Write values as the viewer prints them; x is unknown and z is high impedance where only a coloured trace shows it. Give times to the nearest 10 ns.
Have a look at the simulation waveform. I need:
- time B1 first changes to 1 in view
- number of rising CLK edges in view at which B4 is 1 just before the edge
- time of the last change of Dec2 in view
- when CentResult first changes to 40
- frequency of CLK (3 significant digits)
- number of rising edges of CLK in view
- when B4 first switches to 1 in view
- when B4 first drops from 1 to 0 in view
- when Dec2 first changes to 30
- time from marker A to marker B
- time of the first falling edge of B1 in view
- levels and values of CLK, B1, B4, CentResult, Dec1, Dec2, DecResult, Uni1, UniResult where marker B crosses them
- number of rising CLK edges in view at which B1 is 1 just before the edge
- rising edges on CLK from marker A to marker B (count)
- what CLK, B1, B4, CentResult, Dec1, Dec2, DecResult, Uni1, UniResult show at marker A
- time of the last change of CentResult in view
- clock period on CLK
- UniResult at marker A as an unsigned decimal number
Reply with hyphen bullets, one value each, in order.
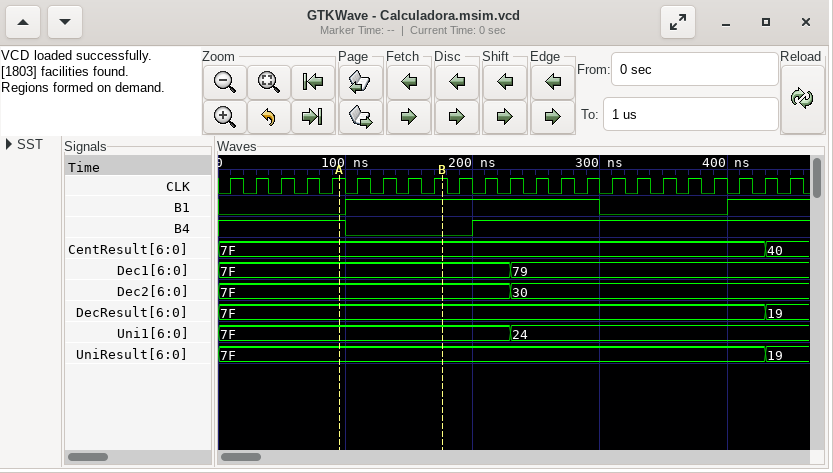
- 100 ns
- 18
- 230 ns
- 430 ns
- 50.0 MHz
- 23
- 200 ns
- 100 ns
- 230 ns
- 80 ns
- 300 ns
- CLK=1, B1=1, B4=0, CentResult=7F, Dec1=7F, Dec2=7F, DecResult=7F, Uni1=7F, UniResult=7F
- 13
- 4
- CLK=1, B1=0, B4=1, CentResult=7F, Dec1=7F, Dec2=7F, DecResult=7F, Uni1=7F, UniResult=7F
- 430 ns
- 20 ns
- 127
